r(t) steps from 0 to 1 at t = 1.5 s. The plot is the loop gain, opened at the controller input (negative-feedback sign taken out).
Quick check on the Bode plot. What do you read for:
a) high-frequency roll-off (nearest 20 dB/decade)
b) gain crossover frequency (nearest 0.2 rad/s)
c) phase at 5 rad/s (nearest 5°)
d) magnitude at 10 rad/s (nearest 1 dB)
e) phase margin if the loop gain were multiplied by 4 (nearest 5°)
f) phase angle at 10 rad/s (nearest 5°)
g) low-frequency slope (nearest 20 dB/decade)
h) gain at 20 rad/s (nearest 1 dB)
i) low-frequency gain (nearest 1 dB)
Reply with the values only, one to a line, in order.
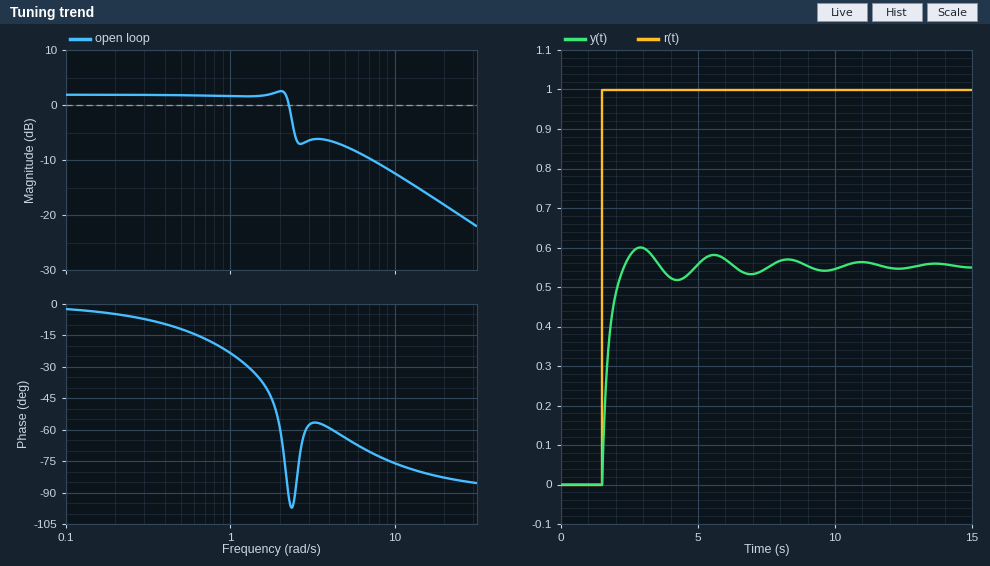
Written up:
-20 dB/decade
2.2 rad/s
-65°
-12 dB
105°
-75°
0 dB/decade
-18 dB
2 dB
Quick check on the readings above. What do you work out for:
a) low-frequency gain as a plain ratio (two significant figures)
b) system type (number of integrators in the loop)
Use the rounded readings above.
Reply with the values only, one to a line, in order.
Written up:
1.3
0
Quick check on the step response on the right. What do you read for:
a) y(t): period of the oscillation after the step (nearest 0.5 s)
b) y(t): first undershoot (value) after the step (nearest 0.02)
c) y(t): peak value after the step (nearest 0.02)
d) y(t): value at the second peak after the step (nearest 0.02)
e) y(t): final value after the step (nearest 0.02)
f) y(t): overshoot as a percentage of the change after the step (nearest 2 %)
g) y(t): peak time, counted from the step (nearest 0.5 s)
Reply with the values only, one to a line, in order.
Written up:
2.5 s
0.52
0.60
0.58
0.56
8 %
1.5 s
